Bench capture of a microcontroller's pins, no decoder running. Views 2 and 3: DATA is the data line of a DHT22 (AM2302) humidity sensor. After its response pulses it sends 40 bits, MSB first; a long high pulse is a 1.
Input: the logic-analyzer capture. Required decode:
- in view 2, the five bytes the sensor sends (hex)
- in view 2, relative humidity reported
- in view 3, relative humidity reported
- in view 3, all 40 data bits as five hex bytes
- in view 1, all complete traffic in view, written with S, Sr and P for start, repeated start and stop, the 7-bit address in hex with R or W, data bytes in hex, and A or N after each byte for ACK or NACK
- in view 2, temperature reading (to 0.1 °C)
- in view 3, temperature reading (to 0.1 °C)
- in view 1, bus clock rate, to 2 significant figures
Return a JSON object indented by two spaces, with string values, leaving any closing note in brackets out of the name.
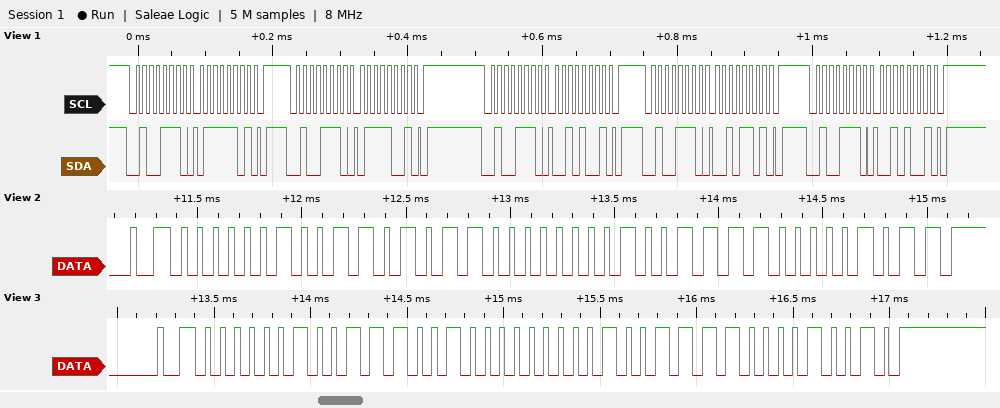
{
  "in view 2, the five bytes the sensor sends": "02 6B 00 9E 0B",
  "in view 2, relative humidity reported": "61.9 %",
  "in view 3, relative humidity reported": "62.6 %",
  "in view 3, all 40 data bits as five hex bytes": "02 72 00 9E 12",
  "in view 1, all complete traffic in view, written with S, Sr and P for start, repeated start and stop, the 7-bit address in hex with R or W, data bytes in hex, and A or N after each byte for ACK or NACK": "S 27W A 7D A P S 27W A 79 A P S 27W A 29 A P S 27W A 2D A P S 27W A 29 A P",
  "in view 2, temperature reading": "15.8 °C",
  "in view 3, temperature reading": "15.8 °C",
  "in view 1, bus clock rate, to 2 significant figures": "100 kHz"
}
